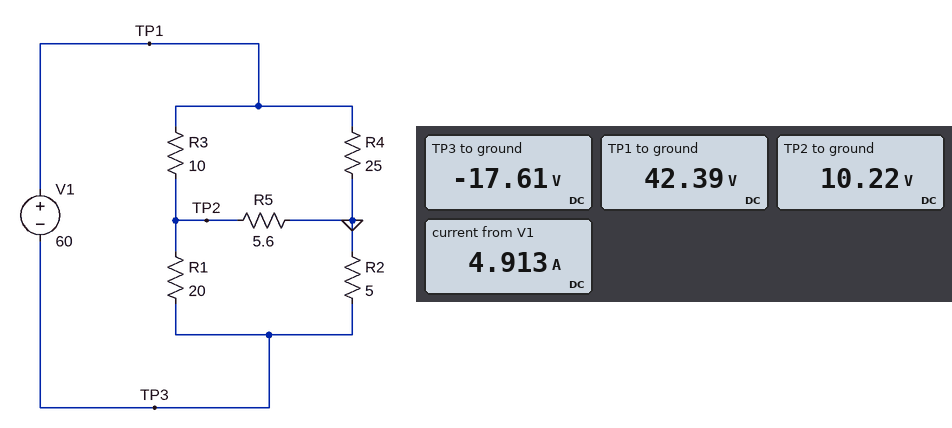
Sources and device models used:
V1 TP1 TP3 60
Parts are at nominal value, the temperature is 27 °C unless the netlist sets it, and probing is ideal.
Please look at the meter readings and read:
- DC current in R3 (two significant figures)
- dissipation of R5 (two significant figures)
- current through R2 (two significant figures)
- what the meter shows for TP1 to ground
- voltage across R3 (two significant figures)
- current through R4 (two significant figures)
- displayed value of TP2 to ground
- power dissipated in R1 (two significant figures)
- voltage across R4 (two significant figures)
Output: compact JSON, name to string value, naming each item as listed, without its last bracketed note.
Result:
{"DC current in R3": "3.2 A", "dissipation of R5": "19 W", "current through R2": "3.5 A", "what the meter shows for TP1 to ground": "42.39 V", "voltage across R3": "32 V", "current through R4": "1.7 A", "displayed value of TP2 to ground": "10.22 V", "power dissipated in R1": "39 W", "voltage across R4": "42 V"}
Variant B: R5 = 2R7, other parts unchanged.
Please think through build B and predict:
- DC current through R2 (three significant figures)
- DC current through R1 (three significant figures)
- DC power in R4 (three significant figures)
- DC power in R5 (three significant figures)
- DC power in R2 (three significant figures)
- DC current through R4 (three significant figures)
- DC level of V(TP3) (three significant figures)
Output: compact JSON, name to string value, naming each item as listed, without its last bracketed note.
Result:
{"DC current through R2": "3.85 A", "DC current through R1": "1.26 A", "DC power in R4": "66.5 W", "DC power in R5": "13.3 W", "DC power in R2": "74.0 W", "DC current through R4": "1.63 A", "DC level of V(TP3)": "-19.2 V"}
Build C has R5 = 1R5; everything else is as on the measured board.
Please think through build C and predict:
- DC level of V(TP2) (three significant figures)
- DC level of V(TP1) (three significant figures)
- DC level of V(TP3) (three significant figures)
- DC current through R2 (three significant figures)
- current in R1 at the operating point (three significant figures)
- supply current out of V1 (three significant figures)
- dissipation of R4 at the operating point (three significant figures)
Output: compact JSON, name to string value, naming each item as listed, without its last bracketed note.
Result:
{"DC level of V(TP2)": "3.65 V", "DC level of V(TP1)": "39.9 V", "DC level of V(TP3)": "-20.1 V", "DC current through R2": "4.03 A", "current in R1 at the operating point": "1.19 A", "supply current out of V1": "5.22 A", "dissipation of R4 at the operating point": "63.6 W"}
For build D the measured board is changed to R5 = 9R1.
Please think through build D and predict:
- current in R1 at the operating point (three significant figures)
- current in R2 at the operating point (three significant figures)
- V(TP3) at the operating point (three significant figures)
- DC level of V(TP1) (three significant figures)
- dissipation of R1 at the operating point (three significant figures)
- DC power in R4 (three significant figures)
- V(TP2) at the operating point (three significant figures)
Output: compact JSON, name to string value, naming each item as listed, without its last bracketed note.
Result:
{"current in R1 at the operating point": "1.50 A", "current in R2 at the operating point": "3.25 A", "V(TP3) at the operating point": "-16.3 V", "DC level of V(TP1)": "43.7 V", "dissipation of R1 at the operating point": "44.9 W", "DC power in R4": "76.5 W", "V(TP2) at the operating point": "13.7 V"}
